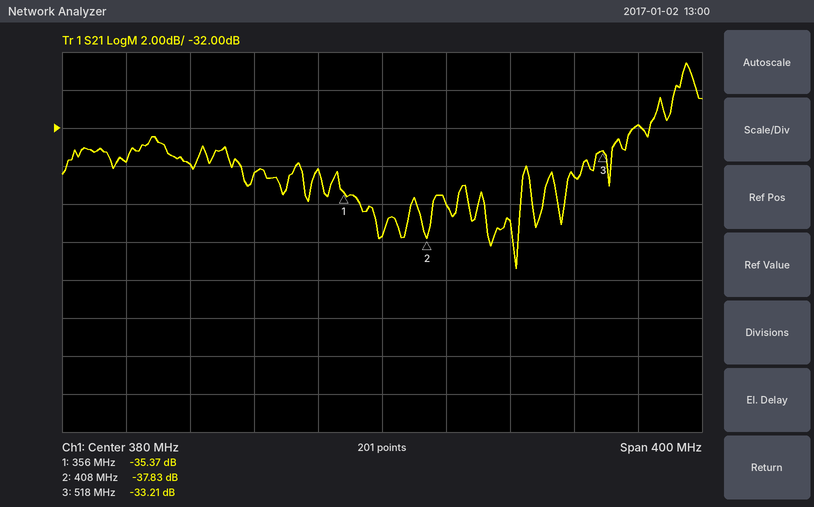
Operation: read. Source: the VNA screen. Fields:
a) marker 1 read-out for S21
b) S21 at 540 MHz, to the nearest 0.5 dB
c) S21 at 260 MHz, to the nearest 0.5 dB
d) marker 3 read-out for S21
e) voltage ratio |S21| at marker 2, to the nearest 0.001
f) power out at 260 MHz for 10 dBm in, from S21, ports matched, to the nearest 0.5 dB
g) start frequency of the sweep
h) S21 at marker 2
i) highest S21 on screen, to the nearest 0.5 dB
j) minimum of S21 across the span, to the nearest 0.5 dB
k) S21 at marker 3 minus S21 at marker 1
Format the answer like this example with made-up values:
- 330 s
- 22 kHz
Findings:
- -35.37 dB
- -32.0 dB
- -34.0 dB
- -33.21 dB
- 0.013
- -24.0 dBm
- 180 MHz
- -37.83 dB
- -28.5 dB
- -39.5 dB
- 2.16 dB
